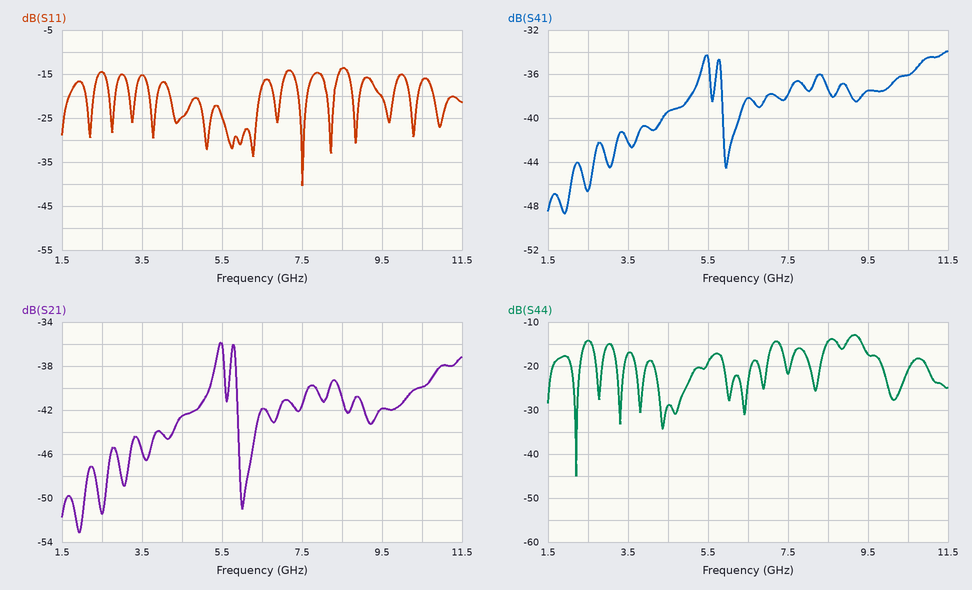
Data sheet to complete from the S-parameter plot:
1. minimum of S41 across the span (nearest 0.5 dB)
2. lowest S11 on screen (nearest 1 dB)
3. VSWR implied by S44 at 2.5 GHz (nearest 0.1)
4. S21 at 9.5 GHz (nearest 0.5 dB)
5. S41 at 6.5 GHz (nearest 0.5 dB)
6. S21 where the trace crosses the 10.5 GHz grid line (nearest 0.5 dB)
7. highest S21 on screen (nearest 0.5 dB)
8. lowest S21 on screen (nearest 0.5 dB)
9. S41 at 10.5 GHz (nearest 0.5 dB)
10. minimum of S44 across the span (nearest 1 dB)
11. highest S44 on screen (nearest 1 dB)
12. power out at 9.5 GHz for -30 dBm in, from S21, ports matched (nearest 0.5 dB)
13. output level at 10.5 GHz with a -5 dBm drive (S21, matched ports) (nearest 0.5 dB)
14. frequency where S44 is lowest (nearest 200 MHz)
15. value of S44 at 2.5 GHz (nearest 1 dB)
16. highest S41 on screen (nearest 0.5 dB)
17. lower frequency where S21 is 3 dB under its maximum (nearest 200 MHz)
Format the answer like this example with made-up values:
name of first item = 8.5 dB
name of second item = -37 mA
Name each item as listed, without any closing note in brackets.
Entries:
minimum of S41 across the span = -48.5 dB
lowest S11 on screen = -40 dB
VSWR implied by S44 at 2.5 GHz = 1.5
S21 at 9.5 GHz = -42.0 dB
S41 at 6.5 GHz = -38.0 dB
S21 where the trace crosses the 10.5 GHz grid line = -40.0 dB
highest S21 on screen = -36.0 dB
lowest S21 on screen = -53.0 dB
S41 at 10.5 GHz = -36.0 dB
minimum of S44 across the span = -45 dB
highest S44 on screen = -13 dB
power out at 9.5 GHz for -30 dBm in, from S21, ports matched = -72.0 dBm
output level at 10.5 GHz with a -5 dBm drive (S21, matched ports) = -45.0 dBm
frequency where S44 is lowest = 2.2 GHz
value of S44 at 2.5 GHz = -14 dB
highest S41 on screen = -34.0 dB
lower frequency where S21 is 3 dB under its maximum = 5.2 GHz
